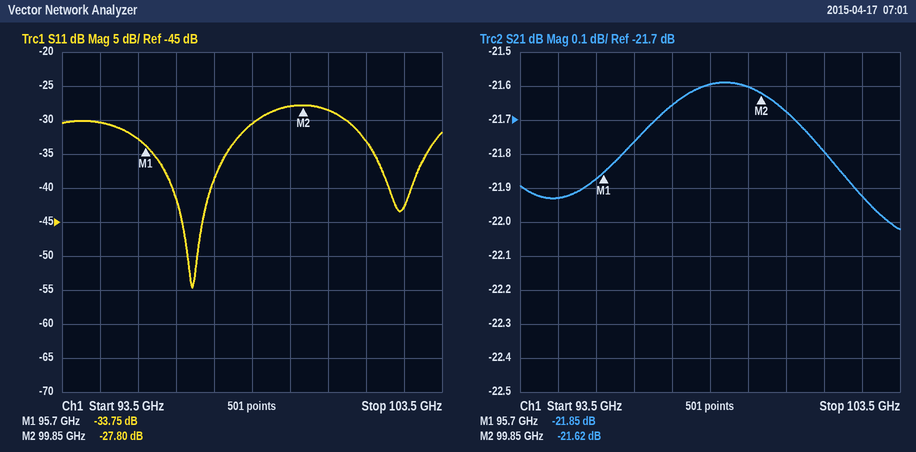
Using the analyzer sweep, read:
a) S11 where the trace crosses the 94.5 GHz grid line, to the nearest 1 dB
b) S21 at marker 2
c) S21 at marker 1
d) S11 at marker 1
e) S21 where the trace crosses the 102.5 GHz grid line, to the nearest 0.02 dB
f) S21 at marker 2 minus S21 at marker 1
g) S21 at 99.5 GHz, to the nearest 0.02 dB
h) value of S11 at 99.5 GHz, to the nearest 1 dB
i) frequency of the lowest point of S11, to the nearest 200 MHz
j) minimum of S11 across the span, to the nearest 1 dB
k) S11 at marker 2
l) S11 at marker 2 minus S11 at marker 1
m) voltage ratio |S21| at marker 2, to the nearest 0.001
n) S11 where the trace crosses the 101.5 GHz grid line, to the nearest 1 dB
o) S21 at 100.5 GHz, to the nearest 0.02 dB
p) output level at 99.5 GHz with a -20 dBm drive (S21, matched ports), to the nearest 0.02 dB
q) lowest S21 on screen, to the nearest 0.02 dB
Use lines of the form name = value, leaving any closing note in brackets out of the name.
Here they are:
S11 where the trace crosses the 94.5 GHz grid line, to the nearest 1 dB = -30 dB
S21 at marker 2 = -21.62 dB
S21 at marker 1 = -21.85 dB
S11 at marker 1 = -33.75 dB
S21 where the trace crosses the 102.5 GHz grid line, to the nearest 0.02 dB = -21.92 dB
S21 at marker 2 minus S21 at marker 1 = 0.23 dB
S21 at 99.5 GHz, to the nearest 0.02 dB = -21.60 dB
value of S11 at 99.5 GHz, to the nearest 1 dB = -28 dB
frequency of the lowest point of S11, to the nearest 200 MHz = 97.0 GHz
minimum of S11 across the span, to the nearest 1 dB = -55 dB
S11 at marker 2 = -27.80 dB
S11 at marker 2 minus S11 at marker 1 = 5.95 dB
voltage ratio |S21| at marker 2, to the nearest 0.001 = 0.083
S11 where the trace crosses the 101.5 GHz grid line, to the nearest 1 dB = -33 dB
S21 at 100.5 GHz, to the nearest 0.02 dB = -21.68 dB
output level at 99.5 GHz with a -20 dBm drive (S21, matched ports), to the nearest 0.02 dB = -41.60 dBm
lowest S21 on screen, to the nearest 0.02 dB = -22.02 dB
